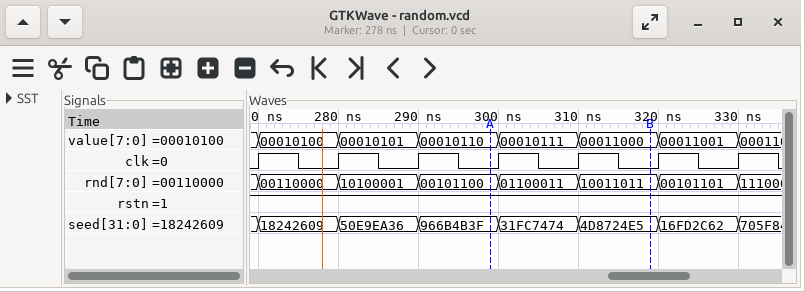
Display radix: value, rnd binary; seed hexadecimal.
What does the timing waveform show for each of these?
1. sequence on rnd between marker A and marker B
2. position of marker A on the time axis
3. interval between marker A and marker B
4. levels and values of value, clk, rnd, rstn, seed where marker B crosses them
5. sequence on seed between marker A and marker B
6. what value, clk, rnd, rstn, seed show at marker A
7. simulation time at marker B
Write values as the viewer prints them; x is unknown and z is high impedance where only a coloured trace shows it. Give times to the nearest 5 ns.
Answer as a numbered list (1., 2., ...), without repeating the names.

1. 00101100, 01100011, 10011011
2. 300 ns
3. 20 ns
4. value=00011000, clk=0, rnd=10011011, rstn=1, seed=4D8724E5
5. 966B4B3F, 31FC7474, 4D8724E5
6. value=00010110, clk=0, rnd=00101100, rstn=1, seed=966B4B3F
7. 320 ns
